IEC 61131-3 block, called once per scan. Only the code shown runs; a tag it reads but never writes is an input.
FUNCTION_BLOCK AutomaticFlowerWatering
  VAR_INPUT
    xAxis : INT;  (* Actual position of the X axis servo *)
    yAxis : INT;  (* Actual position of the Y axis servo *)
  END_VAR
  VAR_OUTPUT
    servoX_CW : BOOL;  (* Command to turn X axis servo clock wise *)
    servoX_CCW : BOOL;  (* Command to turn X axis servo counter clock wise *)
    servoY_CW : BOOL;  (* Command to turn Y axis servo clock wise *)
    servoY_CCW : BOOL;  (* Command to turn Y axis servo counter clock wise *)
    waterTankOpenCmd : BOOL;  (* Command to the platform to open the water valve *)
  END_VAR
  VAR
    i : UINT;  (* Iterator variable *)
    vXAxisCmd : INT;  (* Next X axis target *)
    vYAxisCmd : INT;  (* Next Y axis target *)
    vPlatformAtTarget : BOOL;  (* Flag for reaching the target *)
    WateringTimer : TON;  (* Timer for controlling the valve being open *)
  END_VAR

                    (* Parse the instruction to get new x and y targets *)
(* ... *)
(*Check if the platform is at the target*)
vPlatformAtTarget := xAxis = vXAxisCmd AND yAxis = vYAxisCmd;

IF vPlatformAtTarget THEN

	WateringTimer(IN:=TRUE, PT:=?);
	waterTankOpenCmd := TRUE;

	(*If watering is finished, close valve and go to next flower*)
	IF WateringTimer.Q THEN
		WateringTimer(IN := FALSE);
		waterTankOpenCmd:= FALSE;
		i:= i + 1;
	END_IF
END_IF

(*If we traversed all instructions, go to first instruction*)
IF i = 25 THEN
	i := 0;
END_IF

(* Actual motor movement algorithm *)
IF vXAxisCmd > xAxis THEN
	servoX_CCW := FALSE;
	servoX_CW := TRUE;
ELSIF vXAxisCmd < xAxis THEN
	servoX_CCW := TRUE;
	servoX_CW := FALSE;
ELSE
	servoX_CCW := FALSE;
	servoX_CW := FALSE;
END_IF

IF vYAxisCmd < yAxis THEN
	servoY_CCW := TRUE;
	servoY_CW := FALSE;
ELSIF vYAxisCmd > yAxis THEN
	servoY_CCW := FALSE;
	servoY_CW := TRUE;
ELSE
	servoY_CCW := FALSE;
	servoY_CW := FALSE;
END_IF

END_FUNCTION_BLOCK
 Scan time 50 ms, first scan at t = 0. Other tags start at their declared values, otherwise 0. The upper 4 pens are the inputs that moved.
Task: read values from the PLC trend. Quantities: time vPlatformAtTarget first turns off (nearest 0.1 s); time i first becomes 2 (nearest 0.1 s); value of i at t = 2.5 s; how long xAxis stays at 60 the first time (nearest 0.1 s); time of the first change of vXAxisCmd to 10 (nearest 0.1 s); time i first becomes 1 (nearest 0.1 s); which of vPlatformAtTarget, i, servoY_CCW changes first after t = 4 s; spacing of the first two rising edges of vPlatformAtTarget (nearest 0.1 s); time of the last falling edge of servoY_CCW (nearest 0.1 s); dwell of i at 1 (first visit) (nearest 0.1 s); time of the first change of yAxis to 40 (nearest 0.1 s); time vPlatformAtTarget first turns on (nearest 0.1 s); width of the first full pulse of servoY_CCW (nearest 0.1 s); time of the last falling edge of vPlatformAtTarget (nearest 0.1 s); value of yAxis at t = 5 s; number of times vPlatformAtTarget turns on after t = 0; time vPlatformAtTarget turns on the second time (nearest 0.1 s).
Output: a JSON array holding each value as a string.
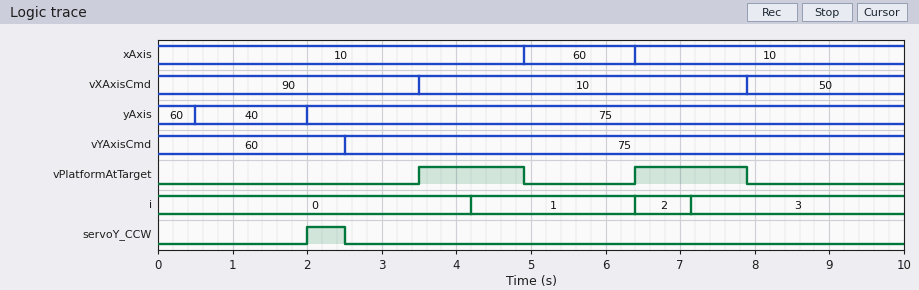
["4.9 s", "6.4 s", "0", "1.5 s", "3.5 s", "4.2 s", "i", "2.9 s", "2.5 s", "2.2 s", "0.5 s", "3.5 s", "0.5 s", "7.9 s", "75", "2", "6.4 s"]
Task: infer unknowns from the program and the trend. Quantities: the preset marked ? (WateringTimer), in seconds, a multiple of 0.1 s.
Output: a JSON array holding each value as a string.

["0.7 s"]
